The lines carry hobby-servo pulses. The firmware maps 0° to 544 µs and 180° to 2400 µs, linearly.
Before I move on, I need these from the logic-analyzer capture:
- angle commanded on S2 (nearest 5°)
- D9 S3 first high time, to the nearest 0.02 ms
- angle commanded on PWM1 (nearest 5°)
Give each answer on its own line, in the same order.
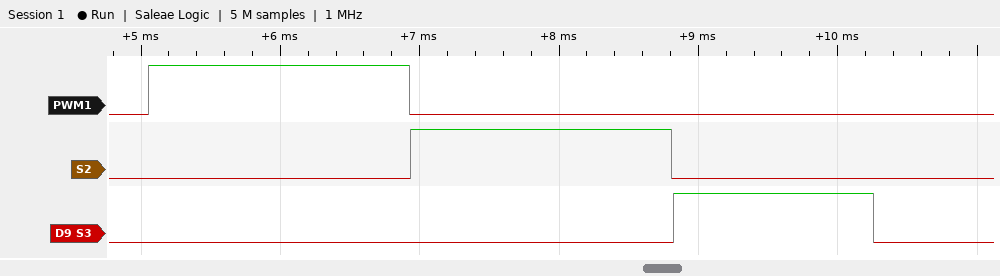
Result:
130°
1.44 ms
130°
